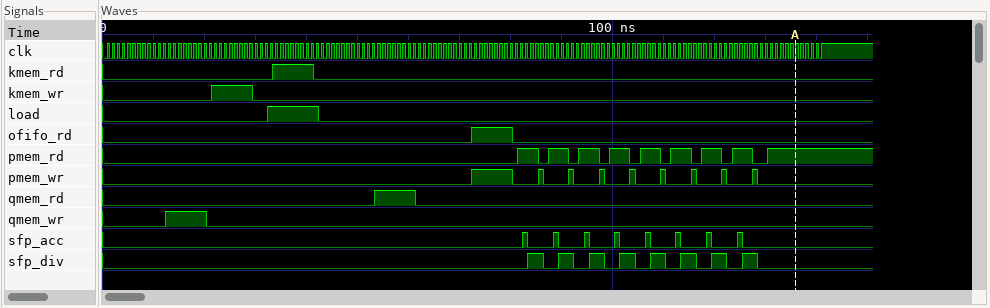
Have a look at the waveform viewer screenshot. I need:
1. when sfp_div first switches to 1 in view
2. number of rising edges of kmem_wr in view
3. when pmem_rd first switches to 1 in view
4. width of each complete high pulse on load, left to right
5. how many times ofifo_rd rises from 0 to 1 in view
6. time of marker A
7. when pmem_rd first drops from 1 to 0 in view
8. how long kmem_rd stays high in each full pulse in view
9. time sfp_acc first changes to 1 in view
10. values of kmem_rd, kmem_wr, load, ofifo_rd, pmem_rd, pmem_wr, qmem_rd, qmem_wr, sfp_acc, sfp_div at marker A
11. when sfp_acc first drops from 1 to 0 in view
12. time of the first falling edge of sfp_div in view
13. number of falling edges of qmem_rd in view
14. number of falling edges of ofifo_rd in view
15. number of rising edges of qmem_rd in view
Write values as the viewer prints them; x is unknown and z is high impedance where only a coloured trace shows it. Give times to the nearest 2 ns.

84 ns
1
82 ns
10 ns
1
136 ns
86 ns
8 ns
82 ns
kmem_rd=0, kmem_wr=0, load=0, ofifo_rd=0, pmem_rd=1, pmem_wr=0, qmem_rd=0, qmem_wr=0, sfp_acc=0, sfp_div=0
84 ns
86 ns
1
1
1
